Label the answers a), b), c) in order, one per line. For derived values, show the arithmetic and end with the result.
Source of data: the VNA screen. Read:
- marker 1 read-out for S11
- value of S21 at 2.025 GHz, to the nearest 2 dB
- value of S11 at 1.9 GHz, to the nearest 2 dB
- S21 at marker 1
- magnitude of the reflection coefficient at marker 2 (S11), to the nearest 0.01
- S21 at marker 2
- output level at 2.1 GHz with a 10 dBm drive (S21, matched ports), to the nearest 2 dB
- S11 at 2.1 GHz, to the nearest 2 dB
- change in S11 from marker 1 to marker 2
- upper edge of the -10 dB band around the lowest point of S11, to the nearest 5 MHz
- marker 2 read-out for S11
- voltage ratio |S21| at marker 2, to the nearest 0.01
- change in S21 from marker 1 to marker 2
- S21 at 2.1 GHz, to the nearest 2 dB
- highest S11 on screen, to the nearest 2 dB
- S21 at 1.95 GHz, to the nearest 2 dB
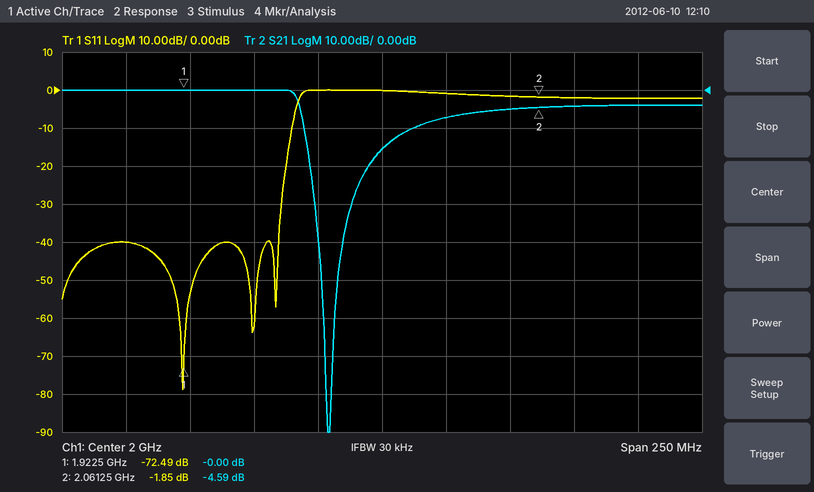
a) -72.49 dB
b) -8 dB
c) -40 dB
d) -0.00 dB
e) 10^(-1.85/20) ≈ 0.81
f) -4.59 dB
g) 10 dBm + (-4 dB) = 6 dBm
h) -2 dB
i) -1.85 − (-72.49) = 70.64 dB
j) 1.965 GHz
k) -1.85 dB
l) 10^(-4.59/20) ≈ 0.59
m) -4.59 − (-0) = -4.59 dB
n) -4 dB
o) 0 dB
p) 0 dB
